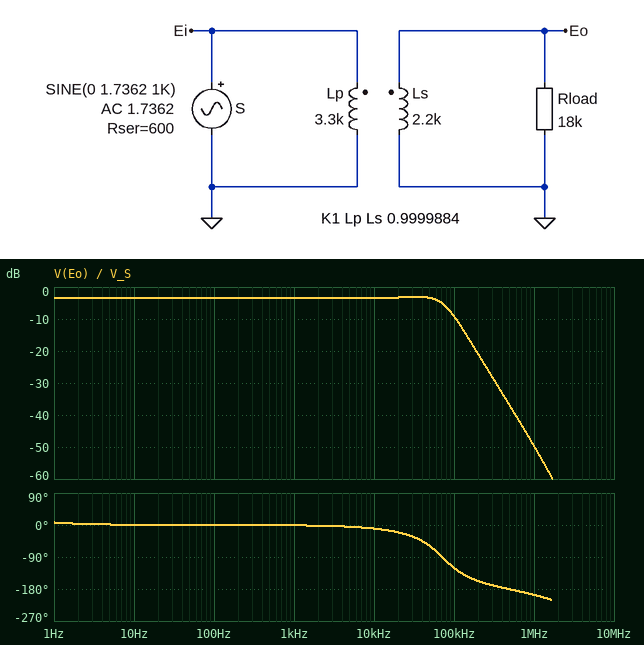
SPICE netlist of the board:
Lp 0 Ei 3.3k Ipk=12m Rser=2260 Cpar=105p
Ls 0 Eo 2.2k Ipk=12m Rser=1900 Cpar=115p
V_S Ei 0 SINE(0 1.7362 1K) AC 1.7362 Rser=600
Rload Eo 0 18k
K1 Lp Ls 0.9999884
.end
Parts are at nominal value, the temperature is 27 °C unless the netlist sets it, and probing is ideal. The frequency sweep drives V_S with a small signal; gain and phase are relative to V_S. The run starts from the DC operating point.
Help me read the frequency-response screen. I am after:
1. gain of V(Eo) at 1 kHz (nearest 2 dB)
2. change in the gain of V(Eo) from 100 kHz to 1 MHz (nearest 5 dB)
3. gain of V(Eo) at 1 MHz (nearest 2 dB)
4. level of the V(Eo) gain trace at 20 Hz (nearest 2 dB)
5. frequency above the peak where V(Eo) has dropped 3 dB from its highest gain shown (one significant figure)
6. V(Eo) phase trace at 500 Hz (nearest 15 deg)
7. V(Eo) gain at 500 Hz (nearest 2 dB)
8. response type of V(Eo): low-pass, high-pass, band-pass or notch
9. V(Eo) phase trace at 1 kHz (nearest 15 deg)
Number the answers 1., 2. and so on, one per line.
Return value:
1. -4 dB
2. -40 dB
3. -50 dB
4. -4 dB
5. 80 kHz
6. 0 deg
7. -4 dB
8. low-pass
9. 0 deg
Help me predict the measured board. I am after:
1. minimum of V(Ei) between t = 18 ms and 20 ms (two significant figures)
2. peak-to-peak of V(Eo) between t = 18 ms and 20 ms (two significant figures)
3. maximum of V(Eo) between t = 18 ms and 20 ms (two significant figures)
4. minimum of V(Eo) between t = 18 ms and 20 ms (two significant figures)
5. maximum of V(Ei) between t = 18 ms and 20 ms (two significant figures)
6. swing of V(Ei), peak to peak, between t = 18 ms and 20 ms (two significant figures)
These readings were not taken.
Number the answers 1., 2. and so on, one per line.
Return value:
1. -1.7 V
2. 2.3 V
3. 1.2 V
4. -1.2 V
5. 1.7 V
6. 3.4 V
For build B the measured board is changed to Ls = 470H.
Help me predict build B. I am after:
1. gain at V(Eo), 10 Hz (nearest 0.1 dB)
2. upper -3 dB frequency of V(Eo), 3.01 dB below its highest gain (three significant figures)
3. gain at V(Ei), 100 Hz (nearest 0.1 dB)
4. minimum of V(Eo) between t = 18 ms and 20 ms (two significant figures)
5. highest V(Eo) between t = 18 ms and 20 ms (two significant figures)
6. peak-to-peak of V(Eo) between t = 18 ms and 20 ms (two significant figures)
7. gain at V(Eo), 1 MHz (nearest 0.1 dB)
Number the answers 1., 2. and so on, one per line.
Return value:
1. -9.5 dB
2. 179 kHz
3. 0 dB
4. -580 mV
5. 580 mV
6. 1.2 V
7. -42.8 dB
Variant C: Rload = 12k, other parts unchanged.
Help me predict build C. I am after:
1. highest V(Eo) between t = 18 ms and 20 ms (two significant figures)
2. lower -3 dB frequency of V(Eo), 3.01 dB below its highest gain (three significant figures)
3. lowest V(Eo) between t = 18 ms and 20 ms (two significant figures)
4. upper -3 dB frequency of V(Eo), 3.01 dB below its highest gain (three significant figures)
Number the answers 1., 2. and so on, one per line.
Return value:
1. 1.1 V
2. 121 mHz
3. -1.1 V
4. 61.4 kHz
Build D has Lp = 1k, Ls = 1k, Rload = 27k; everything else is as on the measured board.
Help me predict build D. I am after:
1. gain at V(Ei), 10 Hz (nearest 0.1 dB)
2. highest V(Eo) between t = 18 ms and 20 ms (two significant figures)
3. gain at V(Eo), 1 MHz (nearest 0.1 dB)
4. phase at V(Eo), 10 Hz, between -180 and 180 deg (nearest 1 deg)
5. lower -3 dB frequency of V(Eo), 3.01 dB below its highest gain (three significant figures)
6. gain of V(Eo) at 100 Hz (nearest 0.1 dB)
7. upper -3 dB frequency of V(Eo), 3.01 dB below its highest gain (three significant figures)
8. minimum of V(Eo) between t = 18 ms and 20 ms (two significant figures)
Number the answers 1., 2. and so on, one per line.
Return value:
1. -0.2 dB
2. 1.5 V
3. -41.0 dB
4. 2 deg
5. 1.65 Hz
6. -1.4 dB
7. 126 kHz
8. -1.5 V
